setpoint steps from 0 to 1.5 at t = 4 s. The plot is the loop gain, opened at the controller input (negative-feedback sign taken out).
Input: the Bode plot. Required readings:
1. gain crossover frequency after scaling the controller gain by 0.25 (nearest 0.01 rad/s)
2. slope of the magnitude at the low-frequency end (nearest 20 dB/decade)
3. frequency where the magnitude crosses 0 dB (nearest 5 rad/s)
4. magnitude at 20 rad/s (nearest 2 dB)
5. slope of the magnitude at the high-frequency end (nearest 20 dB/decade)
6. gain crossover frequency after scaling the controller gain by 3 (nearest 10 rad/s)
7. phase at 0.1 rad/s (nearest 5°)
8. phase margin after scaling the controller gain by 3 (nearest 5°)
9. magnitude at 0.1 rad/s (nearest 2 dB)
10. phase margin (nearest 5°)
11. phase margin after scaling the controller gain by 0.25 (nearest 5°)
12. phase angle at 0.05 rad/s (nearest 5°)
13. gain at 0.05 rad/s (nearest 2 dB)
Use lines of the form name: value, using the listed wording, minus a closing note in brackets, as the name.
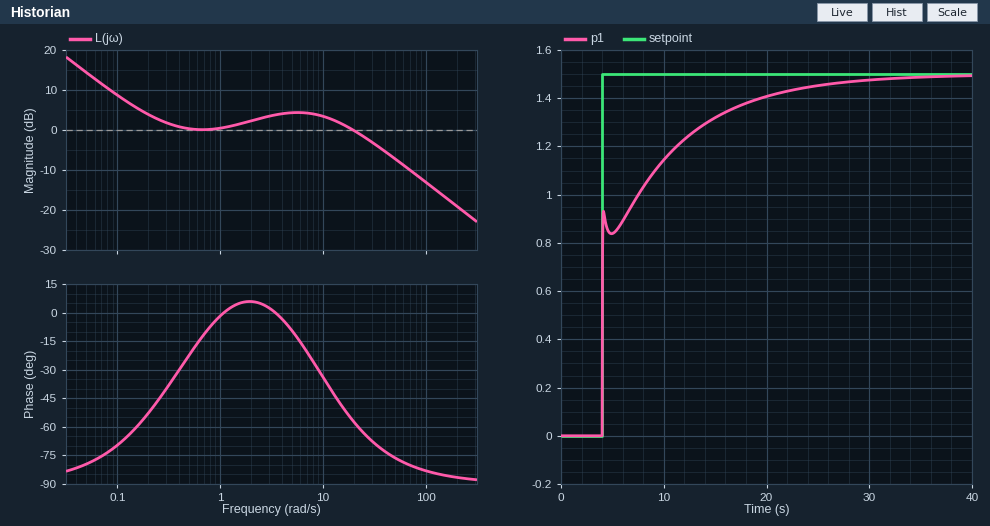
gain crossover frequency after scaling the controller gain by 0.25: 0.07 rad/s
slope of the magnitude at the low-frequency end: -20 dB/decade
frequency where the magnitude crosses 0 dB: 20 rad/s
magnitude at 20 rad/s: 0 dB
slope of the magnitude at the high-frequency end: -20 dB/decade
gain crossover frequency after scaling the controller gain by 3: 70 rad/s
phase at 0.1 rad/s: -70°
phase margin after scaling the controller gain by 3: 100°
magnitude at 0.1 rad/s: 8 dB
phase margin: 125°
phase margin after scaling the controller gain by 0.25: 105°
phase angle at 0.05 rad/s: -80°
gain at 0.05 rad/s: 14 dB
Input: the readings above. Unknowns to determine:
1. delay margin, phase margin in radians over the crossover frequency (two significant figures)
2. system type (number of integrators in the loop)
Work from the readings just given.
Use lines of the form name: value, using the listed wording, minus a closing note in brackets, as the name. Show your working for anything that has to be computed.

delay margin, phase margin in radians over the crossover frequency: 125 × π / 180 / 20 = 0.11 s
system type: 1
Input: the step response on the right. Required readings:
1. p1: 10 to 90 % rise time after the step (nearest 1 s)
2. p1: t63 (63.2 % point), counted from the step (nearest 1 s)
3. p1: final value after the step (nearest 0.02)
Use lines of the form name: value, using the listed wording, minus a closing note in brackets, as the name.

p1: 10 to 90 % rise time after the step: 12 s
p1: t63 (63.2 % point), counted from the step: 3 s
p1: final value after the step: 1.50
